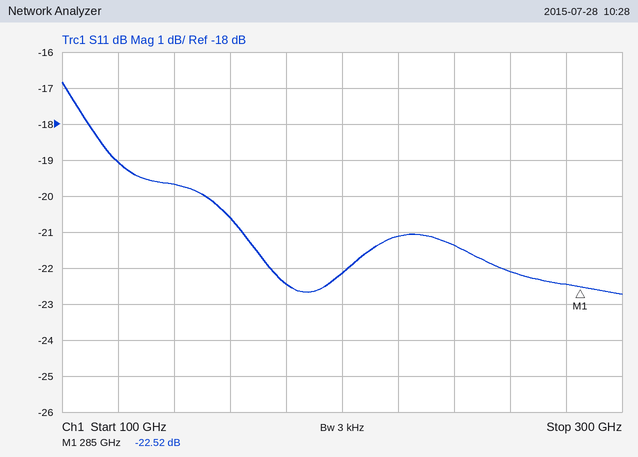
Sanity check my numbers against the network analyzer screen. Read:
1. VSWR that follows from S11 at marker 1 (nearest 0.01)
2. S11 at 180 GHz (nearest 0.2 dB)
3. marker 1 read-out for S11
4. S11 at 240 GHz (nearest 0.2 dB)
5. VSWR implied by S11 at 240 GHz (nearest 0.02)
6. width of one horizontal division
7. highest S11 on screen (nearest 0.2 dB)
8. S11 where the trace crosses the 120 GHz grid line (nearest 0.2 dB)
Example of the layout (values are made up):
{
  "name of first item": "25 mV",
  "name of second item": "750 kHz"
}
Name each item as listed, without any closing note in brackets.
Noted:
{
  "VSWR that follows from S11 at marker 1": "1.16",
  "S11 at 180 GHz": "-22.4 dB",
  "marker 1 read-out for S11": "-22.52 dB",
  "S11 at 240 GHz": "-21.4 dB",
  "VSWR implied by S11 at 240 GHz": "1.18",
  "width of one horizontal division": "20 GHz",
  "highest S11 on screen": "-16.8 dB",
  "S11 where the trace crosses the 120 GHz grid line": "-19.0 dB"
}
